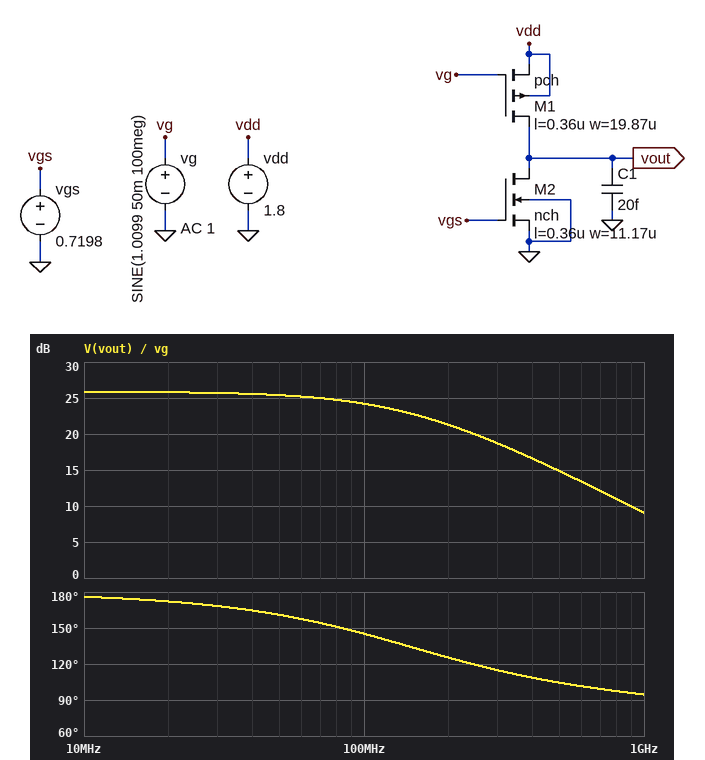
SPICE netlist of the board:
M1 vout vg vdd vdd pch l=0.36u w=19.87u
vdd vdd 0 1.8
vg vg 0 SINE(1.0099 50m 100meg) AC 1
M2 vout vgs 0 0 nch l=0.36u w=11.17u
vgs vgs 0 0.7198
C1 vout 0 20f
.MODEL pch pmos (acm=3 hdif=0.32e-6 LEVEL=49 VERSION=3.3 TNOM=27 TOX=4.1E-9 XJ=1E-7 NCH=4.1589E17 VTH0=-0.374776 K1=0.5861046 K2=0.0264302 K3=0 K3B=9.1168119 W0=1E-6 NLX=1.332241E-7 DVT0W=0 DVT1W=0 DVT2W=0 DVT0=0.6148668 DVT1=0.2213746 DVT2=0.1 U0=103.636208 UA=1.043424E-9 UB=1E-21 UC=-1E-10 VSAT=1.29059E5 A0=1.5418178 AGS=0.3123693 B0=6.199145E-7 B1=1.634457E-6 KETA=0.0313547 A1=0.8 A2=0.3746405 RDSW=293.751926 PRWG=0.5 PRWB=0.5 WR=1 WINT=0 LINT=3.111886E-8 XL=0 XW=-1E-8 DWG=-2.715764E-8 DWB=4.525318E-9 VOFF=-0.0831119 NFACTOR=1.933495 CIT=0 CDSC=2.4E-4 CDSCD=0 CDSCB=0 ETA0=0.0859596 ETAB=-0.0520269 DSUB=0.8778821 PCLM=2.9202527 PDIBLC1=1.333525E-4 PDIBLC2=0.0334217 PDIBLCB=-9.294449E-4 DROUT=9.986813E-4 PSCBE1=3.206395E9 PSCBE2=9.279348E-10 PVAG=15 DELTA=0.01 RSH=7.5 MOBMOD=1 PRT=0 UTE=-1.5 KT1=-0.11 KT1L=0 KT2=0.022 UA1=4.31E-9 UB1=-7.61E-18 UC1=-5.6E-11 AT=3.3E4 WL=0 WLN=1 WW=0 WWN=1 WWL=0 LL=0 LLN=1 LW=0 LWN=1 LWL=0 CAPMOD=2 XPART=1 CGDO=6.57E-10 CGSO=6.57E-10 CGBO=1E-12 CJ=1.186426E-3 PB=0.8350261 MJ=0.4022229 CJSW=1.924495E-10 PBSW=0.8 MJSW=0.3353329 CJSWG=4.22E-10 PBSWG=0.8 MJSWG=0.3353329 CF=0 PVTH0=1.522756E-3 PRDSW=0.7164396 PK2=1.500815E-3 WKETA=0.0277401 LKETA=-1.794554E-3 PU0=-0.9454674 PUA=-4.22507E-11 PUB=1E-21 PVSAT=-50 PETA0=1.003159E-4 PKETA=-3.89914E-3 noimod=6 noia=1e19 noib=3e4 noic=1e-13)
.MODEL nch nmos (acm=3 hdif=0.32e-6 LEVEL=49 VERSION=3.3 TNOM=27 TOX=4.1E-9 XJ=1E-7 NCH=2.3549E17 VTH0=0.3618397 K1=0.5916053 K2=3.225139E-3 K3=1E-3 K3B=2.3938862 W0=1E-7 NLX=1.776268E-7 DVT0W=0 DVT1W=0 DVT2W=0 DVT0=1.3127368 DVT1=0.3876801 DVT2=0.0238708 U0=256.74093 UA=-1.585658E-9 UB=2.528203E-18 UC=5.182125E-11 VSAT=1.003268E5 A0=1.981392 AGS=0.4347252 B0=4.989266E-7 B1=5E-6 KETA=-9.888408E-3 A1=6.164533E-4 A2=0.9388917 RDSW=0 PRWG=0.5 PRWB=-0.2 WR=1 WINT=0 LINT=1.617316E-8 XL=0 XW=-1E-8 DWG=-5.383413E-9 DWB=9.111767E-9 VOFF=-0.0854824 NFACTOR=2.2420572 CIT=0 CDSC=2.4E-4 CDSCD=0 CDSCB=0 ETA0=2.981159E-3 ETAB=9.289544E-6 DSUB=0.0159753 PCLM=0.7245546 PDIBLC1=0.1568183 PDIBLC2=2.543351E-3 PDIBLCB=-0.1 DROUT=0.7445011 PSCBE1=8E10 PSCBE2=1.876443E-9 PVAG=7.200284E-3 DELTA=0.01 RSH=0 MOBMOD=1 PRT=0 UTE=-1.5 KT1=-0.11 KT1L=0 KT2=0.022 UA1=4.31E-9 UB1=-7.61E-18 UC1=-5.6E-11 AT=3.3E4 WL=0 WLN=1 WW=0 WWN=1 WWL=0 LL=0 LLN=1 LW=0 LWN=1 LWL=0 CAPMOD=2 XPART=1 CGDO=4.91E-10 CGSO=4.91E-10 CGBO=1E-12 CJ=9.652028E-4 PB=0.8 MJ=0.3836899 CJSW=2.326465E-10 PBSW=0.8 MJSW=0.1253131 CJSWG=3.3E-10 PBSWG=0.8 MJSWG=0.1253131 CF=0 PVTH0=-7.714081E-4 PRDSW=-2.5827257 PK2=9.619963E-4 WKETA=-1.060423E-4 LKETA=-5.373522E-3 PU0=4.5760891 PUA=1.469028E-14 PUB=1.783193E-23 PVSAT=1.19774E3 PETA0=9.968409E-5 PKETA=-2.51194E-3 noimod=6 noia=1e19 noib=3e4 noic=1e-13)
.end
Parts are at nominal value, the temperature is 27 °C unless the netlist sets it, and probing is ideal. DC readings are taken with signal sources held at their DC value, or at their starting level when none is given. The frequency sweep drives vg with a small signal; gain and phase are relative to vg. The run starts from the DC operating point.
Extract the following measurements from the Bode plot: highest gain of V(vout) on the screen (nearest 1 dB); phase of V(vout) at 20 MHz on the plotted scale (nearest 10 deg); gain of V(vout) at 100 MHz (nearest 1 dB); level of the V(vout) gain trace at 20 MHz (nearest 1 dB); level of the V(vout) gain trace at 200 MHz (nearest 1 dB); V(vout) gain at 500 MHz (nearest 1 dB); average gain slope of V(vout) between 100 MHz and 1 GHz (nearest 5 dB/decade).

26 dB
170 deg
24 dB
26 dB
21 dB
15 dB
-15 dB/decade
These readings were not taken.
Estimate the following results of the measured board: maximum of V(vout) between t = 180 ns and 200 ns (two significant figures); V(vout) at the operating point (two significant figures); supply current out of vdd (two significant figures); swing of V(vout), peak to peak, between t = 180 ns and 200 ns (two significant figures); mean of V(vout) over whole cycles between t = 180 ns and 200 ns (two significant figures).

1.3 V
410 mV
240 µA
1.2 V
620 mV
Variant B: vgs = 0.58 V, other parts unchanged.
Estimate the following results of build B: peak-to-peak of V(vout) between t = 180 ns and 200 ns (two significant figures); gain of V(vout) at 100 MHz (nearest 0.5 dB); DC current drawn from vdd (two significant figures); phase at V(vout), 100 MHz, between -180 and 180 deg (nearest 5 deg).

19 mV
-14.5 dB
66 µA
170 deg
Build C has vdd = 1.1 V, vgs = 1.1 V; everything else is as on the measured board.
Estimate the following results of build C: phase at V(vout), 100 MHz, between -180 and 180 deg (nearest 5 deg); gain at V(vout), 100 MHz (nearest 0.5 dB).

90 deg
-57.5 dB
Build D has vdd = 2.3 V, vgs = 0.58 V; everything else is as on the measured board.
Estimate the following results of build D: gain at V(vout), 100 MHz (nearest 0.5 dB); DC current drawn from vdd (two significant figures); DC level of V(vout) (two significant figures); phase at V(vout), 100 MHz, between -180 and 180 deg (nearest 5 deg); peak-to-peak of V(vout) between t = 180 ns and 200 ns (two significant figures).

-32.5 dB
72 µA
2.3 V
160 deg
2.4 mV
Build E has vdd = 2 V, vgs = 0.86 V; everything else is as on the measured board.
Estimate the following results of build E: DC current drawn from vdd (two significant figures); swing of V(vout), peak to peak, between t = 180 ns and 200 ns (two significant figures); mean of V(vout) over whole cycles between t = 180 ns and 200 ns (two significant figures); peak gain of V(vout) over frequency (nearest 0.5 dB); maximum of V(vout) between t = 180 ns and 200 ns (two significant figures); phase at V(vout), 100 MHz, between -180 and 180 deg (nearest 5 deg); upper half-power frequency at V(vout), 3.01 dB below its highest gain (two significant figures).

550 µA
1.0 V
600 mV
21.0 dB
1.2 V
165 deg
350 MHz
